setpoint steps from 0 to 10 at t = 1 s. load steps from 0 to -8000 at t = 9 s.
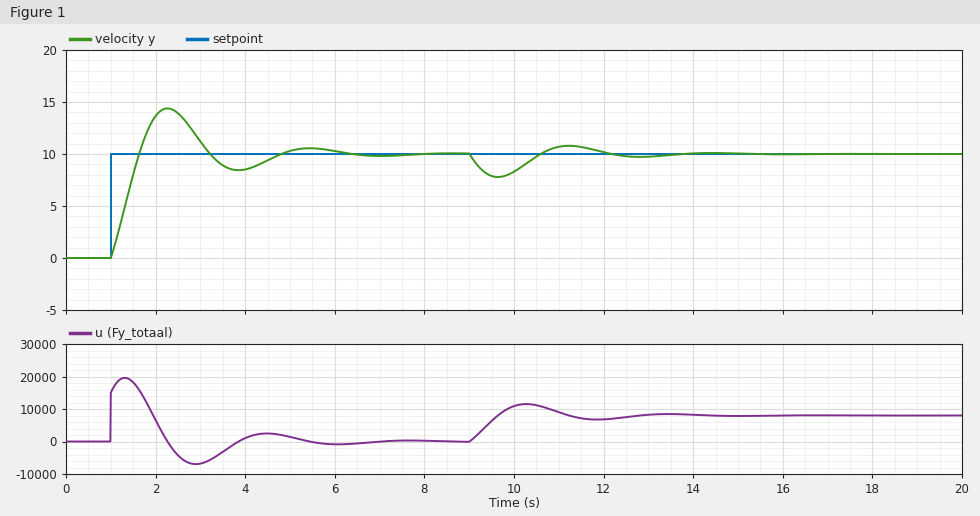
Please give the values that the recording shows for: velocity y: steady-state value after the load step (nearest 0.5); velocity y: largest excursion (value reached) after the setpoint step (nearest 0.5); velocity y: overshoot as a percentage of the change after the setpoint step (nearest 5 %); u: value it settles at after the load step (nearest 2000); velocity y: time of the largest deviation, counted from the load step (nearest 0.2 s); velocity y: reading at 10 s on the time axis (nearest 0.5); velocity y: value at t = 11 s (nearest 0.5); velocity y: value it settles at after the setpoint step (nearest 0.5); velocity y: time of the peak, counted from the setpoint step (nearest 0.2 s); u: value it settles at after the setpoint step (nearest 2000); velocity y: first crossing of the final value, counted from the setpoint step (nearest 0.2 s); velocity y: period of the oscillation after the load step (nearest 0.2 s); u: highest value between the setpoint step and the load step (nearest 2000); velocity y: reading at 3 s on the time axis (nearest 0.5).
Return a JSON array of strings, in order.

["10.0", "14.5", "45 %", "8000", "0.6 s", "8.5", "10.5", "10.0", "1.2 s", "0", "0.6 s", "3.2 s", "20000", "11.0"]
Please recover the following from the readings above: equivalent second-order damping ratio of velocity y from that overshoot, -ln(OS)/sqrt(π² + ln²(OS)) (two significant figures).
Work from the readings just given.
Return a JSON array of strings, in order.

["0.25"]
